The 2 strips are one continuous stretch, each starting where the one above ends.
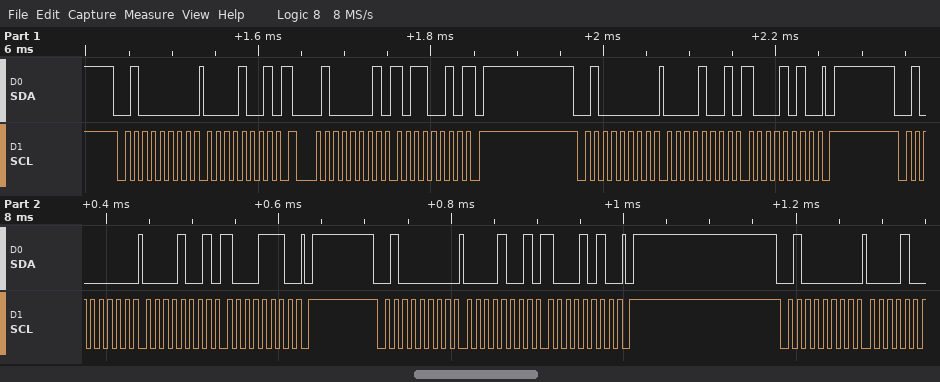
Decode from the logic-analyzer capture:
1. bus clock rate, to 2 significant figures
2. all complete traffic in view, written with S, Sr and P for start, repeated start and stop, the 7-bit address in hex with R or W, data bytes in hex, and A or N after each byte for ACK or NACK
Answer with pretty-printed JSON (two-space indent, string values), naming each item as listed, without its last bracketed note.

{
  "bus clock rate, to 2 significant figures": "100 kHz",
  "all complete traffic in view, written with S, Sr and P for start, repeated start and stop, the 7-bit address in hex with R or W, data bytes in hex, and A or N after each byte for ACK or NACK": "S 20W A 09 A Sr 20R A B2 N P S 20W A 09 A 8A A P S 20W A 09 A 8E A P S 20W A 09 A 8A A P S 20W A"
}
